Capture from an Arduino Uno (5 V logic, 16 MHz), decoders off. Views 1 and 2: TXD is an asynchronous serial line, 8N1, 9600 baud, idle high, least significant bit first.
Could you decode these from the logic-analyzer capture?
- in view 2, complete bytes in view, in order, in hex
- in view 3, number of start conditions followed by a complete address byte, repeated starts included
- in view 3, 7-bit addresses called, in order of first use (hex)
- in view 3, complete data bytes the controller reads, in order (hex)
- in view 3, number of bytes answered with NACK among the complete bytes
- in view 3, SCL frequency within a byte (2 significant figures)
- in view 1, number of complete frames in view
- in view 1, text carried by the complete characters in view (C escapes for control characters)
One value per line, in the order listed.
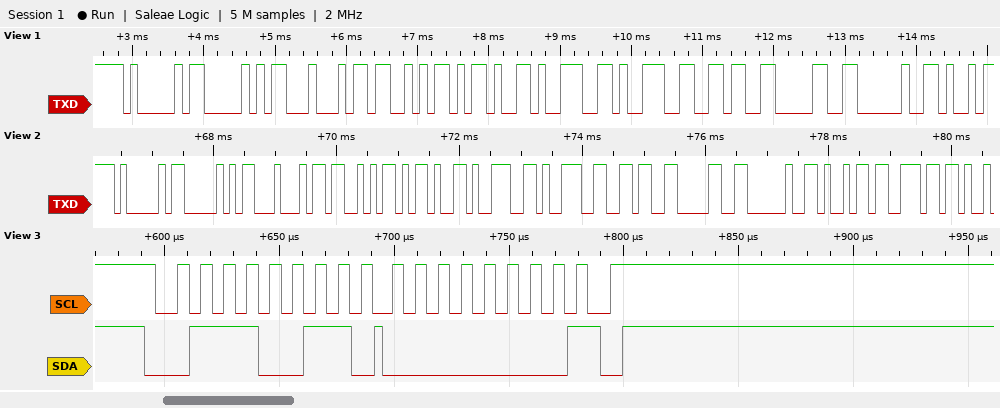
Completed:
41 50 44 53 2D 39 39 36 30 20 69 6E
1
0x39
00
1
100 kHz
10
"APDS-9960 "
